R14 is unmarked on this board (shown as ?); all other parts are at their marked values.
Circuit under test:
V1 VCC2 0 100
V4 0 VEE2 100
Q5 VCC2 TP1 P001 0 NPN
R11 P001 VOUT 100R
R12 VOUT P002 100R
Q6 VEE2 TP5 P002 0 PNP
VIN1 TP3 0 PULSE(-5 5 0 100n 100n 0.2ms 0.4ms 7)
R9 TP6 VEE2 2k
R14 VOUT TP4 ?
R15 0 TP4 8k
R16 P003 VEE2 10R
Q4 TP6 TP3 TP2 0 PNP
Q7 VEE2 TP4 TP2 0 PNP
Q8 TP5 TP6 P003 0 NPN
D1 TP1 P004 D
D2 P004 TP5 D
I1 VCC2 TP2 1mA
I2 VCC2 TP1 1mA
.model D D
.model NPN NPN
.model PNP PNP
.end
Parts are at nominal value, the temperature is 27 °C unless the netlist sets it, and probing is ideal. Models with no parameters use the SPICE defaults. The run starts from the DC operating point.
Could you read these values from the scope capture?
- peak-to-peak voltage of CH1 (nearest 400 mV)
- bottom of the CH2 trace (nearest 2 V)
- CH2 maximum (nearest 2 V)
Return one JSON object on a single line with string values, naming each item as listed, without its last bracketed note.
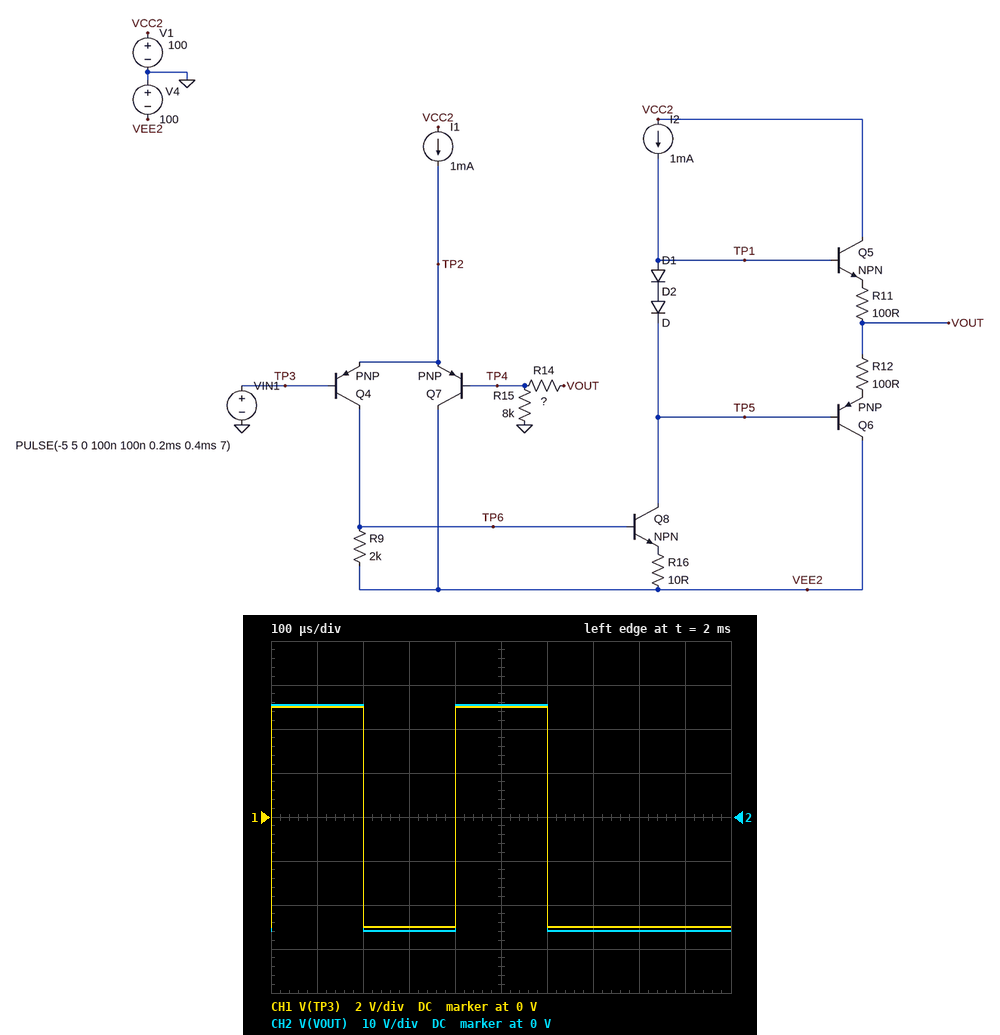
{"peak-to-peak voltage of CH1": "10.0 V", "bottom of the CH2 trace": "-26 V", "CH2 maximum": "26 V"}
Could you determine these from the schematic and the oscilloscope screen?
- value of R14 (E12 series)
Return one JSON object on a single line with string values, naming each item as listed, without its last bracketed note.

{"value of R14": "33 kΩ"}
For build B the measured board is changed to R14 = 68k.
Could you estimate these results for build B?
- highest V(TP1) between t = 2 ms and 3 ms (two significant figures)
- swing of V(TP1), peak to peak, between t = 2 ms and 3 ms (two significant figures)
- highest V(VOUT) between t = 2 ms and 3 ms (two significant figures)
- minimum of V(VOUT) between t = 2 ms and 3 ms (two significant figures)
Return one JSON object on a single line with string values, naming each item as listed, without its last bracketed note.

{"highest V(TP1) between t = 2 ms and 3 ms": "48 V", "swing of V(TP1), peak to peak, between t = 2 ms and 3 ms": "95 V", "highest V(VOUT) between t = 2 ms and 3 ms": "47 V", "minimum of V(VOUT) between t = 2 ms and 3 ms": "-48 V"}
